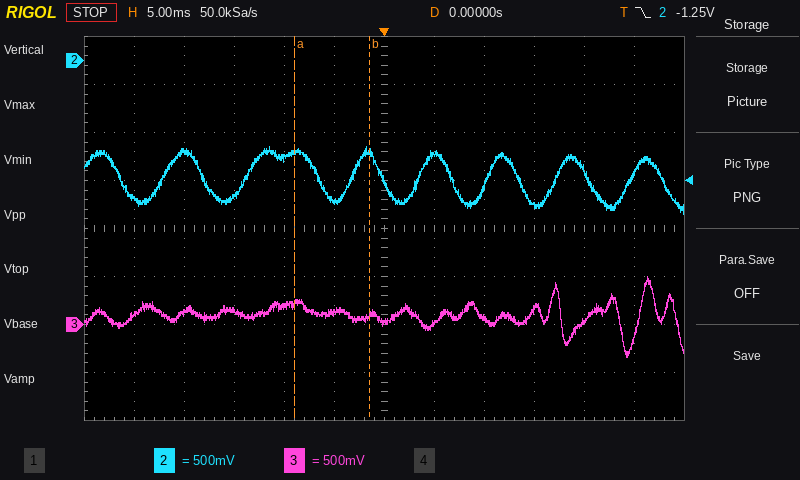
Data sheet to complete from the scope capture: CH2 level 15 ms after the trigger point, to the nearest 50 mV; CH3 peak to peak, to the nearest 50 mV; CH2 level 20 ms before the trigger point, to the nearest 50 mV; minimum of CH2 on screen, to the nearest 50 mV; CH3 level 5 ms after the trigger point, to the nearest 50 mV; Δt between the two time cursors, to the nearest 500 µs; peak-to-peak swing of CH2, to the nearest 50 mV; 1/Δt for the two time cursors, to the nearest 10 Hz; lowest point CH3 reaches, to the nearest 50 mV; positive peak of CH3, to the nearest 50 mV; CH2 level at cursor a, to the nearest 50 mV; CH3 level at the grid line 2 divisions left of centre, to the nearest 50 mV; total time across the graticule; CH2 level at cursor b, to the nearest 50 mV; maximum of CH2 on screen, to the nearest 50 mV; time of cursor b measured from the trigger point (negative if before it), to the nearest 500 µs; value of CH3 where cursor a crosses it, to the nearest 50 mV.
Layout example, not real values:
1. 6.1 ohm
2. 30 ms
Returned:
1. -1.50 V
2. 850 mV
3. -950 mV
4. -1.60 V
5. 0 mV
6. 7.5 ms
7. 700 mV
8. 130 Hz
9. -350 mV
10. 500 mV
11. -950 mV
12. 200 mV
13. 60 ms
14. -950 mV
15. -900 mV
16. -1.5 ms
17. 200 mV
